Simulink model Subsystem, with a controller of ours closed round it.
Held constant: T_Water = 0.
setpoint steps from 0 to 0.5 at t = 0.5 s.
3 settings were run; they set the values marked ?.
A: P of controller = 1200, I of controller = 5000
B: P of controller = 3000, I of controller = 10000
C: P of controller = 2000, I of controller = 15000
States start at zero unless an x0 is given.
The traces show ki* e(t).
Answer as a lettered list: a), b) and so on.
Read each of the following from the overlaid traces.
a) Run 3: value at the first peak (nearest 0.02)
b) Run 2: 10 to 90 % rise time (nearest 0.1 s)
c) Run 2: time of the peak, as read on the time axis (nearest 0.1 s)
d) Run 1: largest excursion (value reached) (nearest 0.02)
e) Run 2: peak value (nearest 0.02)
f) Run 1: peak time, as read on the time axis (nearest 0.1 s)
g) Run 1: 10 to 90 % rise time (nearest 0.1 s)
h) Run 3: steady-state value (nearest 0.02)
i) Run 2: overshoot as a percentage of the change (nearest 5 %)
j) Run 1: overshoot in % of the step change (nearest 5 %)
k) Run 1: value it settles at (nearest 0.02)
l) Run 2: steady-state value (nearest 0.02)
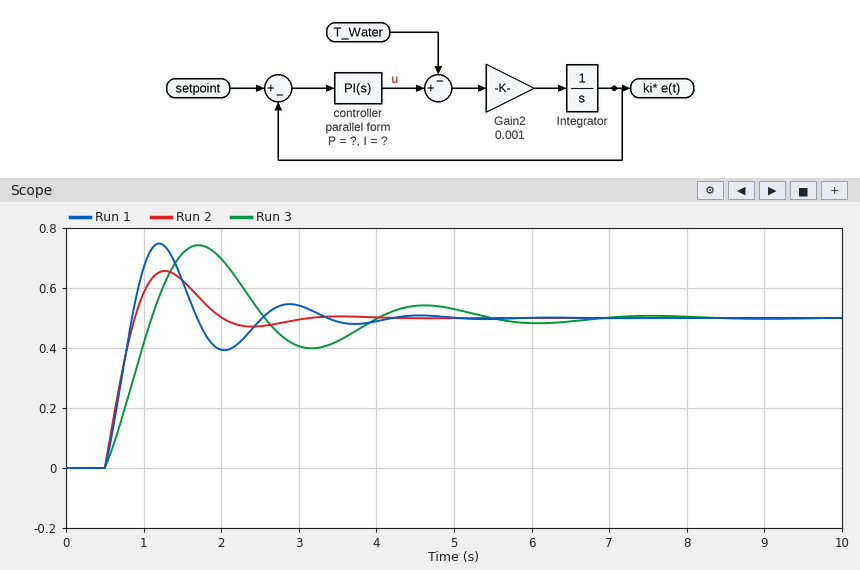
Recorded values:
a) 0.74
b) 0.3 s
c) 1.3 s
d) 0.74
e) 0.66
f) 1.2 s
g) 0.3 s
h) 0.50
i) 30 %
j) 50 %
k) 0.50
l) 0.50
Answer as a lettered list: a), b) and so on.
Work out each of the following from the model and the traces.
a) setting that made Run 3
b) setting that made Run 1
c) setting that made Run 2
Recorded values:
a) A
b) C
c) B
